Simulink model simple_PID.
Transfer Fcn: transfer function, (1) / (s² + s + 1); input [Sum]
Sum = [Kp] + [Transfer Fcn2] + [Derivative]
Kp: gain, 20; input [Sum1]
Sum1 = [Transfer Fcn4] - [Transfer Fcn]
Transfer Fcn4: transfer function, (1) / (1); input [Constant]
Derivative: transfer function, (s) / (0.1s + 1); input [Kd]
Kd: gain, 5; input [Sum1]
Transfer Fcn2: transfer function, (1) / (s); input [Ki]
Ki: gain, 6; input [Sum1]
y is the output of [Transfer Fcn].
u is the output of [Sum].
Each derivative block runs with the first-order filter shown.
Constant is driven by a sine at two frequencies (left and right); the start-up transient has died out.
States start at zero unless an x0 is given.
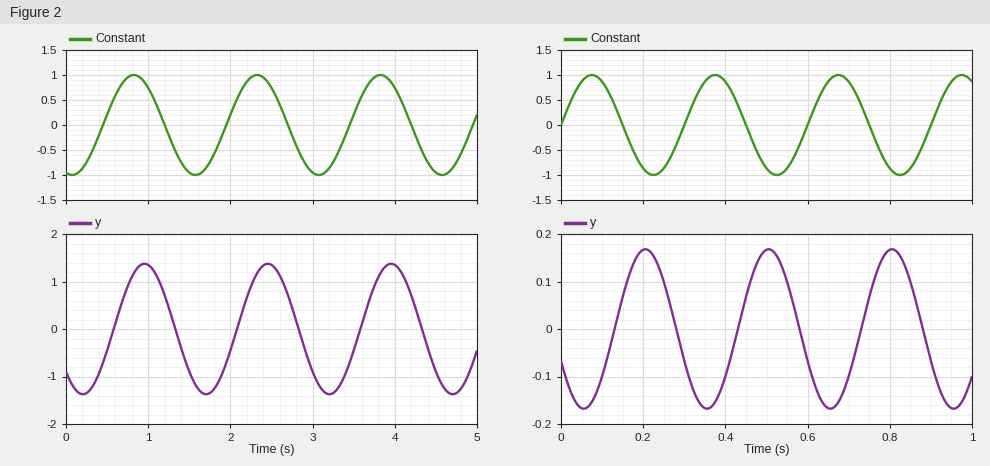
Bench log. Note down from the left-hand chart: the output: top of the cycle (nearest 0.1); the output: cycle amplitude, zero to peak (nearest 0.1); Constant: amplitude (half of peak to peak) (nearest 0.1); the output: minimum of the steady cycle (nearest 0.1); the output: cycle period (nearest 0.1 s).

1.4
1.4
1.0
-1.4
1.5 s
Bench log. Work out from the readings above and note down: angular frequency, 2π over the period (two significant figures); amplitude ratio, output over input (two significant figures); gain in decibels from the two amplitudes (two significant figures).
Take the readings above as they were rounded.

4.2 rad/s
1.4
2.9 dB
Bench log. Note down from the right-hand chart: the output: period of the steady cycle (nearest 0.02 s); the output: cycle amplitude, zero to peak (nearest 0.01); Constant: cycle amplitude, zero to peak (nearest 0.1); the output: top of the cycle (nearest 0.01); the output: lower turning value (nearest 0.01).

0.30 s
0.17
1.0
0.17
-0.17
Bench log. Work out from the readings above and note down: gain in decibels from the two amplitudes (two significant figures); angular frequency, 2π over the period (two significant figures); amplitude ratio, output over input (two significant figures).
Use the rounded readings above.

-15 dB
21 rad/s
0.17
